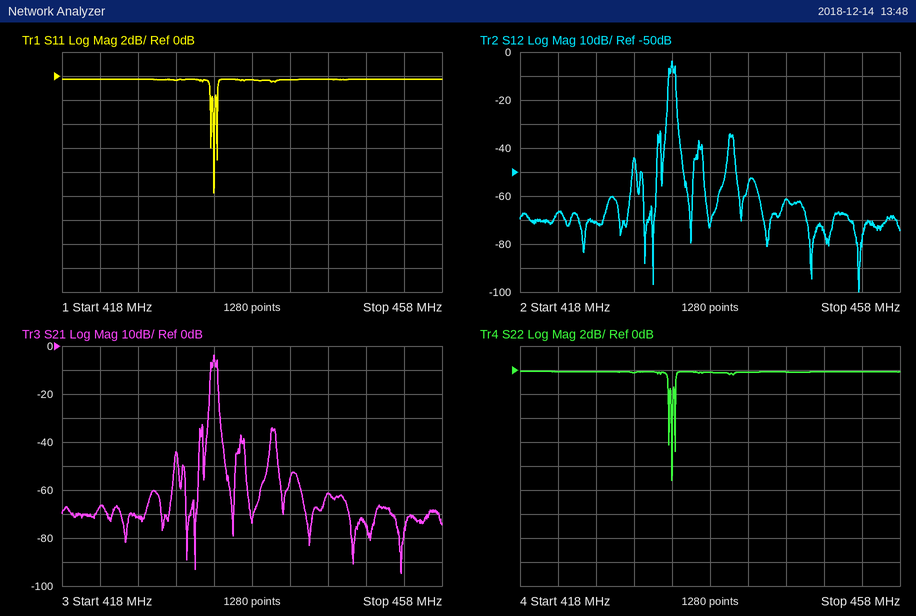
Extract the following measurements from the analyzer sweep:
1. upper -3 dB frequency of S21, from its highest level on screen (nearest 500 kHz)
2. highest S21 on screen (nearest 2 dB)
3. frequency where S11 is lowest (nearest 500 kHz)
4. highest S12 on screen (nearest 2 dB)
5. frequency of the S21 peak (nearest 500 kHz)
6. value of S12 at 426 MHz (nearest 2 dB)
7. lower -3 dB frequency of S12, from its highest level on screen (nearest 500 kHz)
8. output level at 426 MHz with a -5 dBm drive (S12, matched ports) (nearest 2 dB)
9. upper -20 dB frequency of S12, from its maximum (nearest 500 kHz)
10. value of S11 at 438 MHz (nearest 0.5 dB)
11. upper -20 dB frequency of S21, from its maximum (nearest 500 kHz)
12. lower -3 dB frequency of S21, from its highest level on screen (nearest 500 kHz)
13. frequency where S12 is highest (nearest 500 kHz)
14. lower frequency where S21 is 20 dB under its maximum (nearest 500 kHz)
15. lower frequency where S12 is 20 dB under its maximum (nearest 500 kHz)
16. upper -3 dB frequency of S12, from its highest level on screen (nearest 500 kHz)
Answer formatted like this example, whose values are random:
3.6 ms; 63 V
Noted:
434.0 MHz; -4 dB; 434.0 MHz; -4 dB; 434.0 MHz; -70 dB; 434.0 MHz; -76 dBm; 434.5 MHz; -0.5 dB; 434.5 MHz; 434.0 MHz; 434.0 MHz; 433.5 MHz; 433.5 MHz; 434.0 MHz
